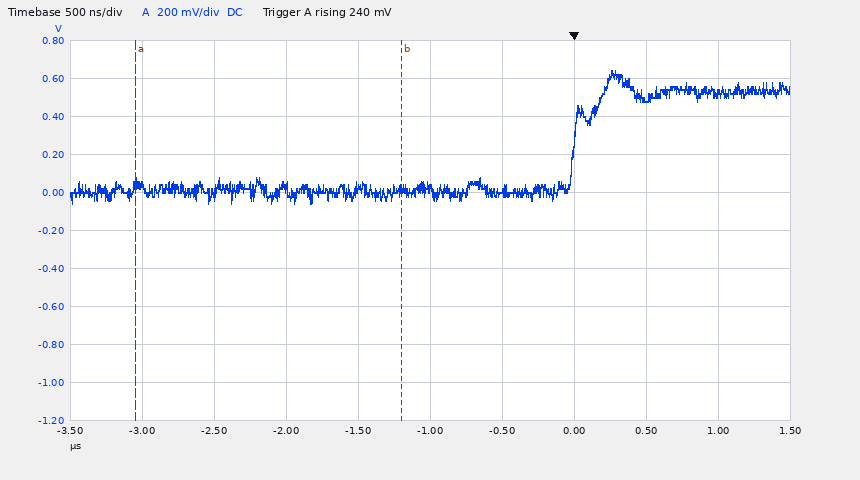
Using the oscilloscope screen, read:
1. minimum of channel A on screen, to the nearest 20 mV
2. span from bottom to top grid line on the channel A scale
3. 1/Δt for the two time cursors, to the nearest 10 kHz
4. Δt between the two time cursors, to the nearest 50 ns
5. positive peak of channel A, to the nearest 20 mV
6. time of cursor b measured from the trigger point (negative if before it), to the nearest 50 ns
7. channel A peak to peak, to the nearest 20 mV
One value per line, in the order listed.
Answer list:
-60 mV
2 V
540 kHz
1.85 µs
640 mV
-1.20 µs
700 mV
